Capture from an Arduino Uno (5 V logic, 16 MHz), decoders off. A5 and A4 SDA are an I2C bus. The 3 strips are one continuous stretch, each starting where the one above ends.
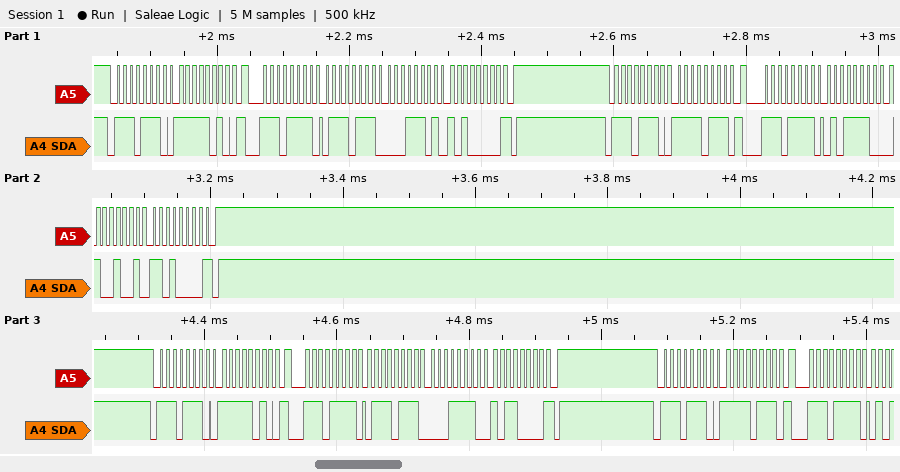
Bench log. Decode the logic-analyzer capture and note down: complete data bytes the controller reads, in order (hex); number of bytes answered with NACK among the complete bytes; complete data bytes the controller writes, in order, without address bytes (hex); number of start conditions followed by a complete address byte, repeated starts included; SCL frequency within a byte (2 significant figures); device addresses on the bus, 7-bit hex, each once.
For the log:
77 1D A0 5E 49 D0 77 1E B0
3
FA F7 FA F7
8
100 kHz
0x77
